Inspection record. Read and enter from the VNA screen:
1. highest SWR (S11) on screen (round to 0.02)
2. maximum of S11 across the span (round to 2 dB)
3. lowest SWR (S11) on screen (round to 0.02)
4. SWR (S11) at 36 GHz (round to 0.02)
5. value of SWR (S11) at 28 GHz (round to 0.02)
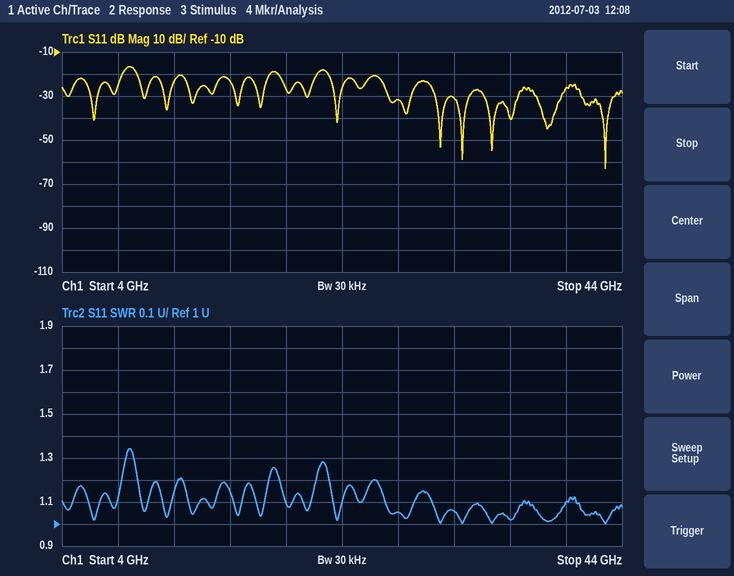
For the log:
1.34
-16 dB
1.00
1.02
1.06
